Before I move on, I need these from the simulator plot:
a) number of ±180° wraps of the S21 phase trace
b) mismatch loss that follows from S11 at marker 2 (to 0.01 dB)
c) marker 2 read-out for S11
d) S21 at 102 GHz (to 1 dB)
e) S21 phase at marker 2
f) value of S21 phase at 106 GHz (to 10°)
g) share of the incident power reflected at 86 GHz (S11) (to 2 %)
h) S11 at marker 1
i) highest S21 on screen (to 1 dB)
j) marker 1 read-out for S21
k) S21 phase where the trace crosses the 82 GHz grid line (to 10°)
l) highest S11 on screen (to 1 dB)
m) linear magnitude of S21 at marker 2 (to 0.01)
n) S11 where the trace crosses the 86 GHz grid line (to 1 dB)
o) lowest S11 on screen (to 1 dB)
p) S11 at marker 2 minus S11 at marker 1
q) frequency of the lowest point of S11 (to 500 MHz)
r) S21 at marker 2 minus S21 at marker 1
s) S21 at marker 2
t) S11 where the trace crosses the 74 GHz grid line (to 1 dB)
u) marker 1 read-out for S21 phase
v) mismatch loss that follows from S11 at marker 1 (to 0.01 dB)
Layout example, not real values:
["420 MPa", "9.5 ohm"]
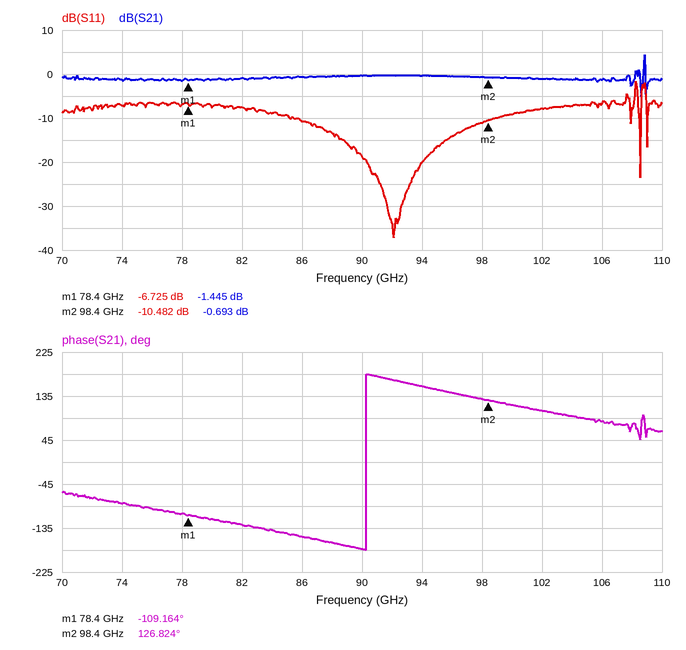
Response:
["1", "0.41 dB", "-10.482 dB", "-1 dB", "126.824°", "80°", "8 %", "-6.725 dB", "4 dB", "-1.445 dB", "-130°", "-2 dB", "0.92", "-11 dB", "-37 dB", "-3.757 dB", "92.0 GHz", "0.752 dB", "-0.693 dB", "-7 dB", "-109.164°", "1.04 dB"]
